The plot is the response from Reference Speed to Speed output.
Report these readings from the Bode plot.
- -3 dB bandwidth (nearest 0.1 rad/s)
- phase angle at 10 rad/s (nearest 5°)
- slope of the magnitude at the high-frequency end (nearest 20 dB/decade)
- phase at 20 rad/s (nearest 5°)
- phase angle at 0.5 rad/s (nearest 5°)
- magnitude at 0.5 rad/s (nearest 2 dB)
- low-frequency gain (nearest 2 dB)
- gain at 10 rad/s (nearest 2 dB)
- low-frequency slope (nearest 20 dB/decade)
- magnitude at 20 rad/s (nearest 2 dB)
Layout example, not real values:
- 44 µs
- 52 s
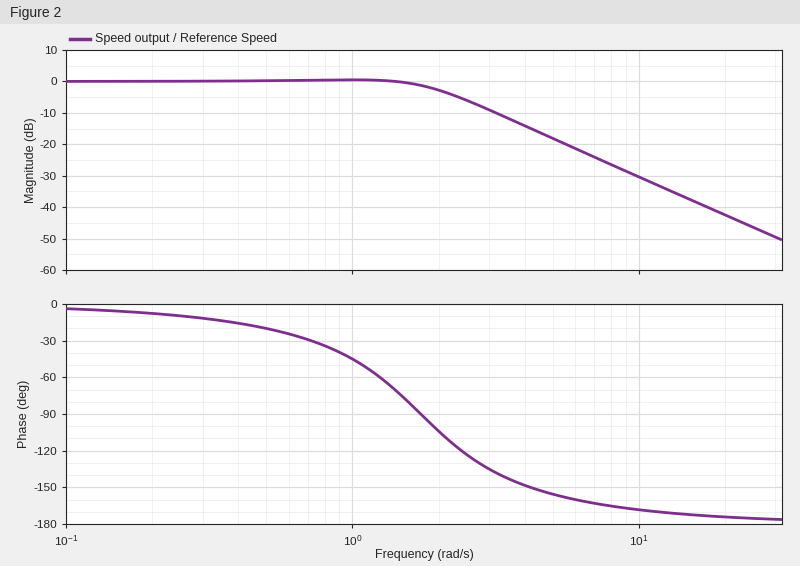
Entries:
- 2.0 rad/s
- -170°
- -40 dB/decade
- -175°
- -20°
- 0 dB
- 0 dB
- -30 dB
- 0 dB/decade
- -42 dB
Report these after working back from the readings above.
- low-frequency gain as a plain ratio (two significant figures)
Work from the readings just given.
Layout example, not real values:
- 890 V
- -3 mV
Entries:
- 1.0
